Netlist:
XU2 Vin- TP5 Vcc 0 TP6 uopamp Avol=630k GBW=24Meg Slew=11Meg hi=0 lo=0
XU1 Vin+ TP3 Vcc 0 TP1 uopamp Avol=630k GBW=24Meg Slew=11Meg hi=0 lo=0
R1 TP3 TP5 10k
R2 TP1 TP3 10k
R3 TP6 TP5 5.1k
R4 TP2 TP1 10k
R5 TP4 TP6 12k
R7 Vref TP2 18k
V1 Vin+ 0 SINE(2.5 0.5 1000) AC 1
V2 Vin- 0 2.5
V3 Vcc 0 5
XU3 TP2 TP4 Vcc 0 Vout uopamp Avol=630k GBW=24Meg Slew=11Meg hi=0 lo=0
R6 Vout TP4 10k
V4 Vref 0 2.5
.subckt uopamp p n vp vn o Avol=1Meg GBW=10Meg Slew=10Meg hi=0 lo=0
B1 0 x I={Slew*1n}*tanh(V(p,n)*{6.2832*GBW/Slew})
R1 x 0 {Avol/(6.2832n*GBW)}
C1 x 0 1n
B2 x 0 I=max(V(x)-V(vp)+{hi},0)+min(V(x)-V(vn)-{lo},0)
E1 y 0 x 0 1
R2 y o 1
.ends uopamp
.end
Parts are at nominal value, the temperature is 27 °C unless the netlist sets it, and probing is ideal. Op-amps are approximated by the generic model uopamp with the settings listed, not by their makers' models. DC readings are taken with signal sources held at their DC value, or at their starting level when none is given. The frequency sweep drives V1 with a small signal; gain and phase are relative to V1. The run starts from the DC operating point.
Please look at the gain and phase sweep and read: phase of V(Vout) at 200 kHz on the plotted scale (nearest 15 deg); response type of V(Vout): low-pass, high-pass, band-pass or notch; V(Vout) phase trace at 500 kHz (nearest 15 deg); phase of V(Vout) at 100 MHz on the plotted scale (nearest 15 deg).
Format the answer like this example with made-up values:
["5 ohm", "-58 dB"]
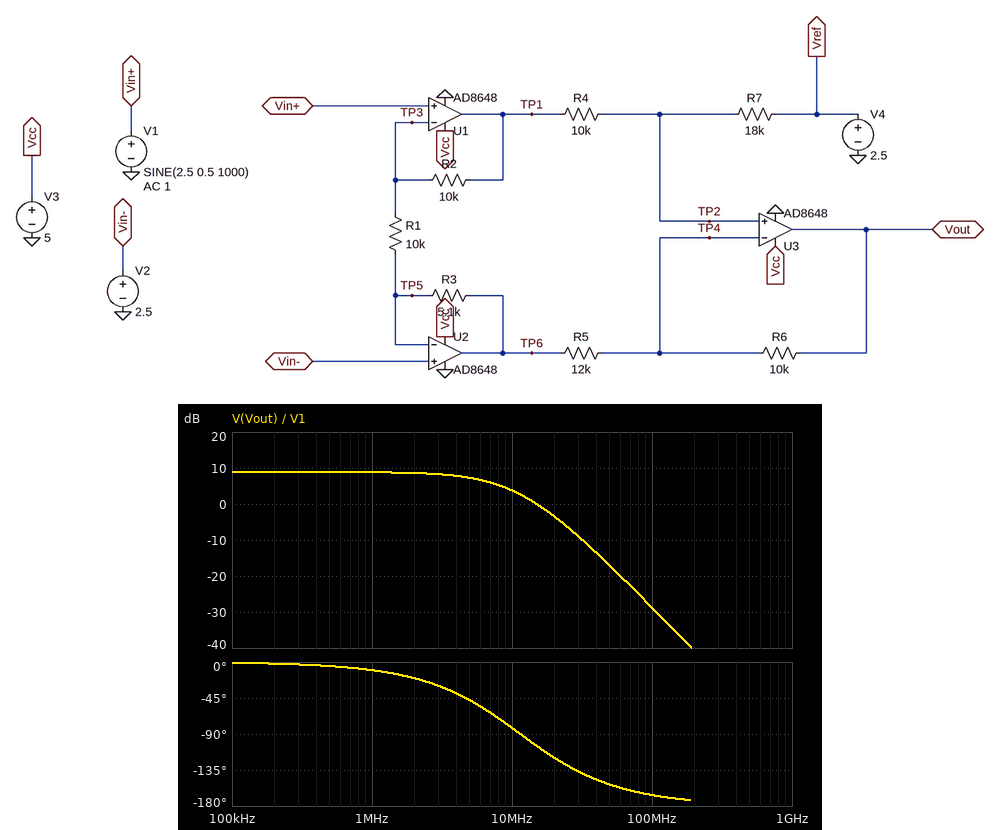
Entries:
["0 deg", "low-pass", "0 deg", "-165 deg"]
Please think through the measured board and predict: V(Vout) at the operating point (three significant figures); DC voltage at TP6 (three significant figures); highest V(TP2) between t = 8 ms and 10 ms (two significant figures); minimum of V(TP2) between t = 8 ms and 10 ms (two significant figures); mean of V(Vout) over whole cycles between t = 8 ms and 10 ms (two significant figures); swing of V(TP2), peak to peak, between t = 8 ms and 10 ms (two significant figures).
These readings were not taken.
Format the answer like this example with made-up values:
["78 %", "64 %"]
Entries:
["2.50 V", "2.50 V", "3.1 V", "1.9 V", "2.5 V", "1.3 V"]
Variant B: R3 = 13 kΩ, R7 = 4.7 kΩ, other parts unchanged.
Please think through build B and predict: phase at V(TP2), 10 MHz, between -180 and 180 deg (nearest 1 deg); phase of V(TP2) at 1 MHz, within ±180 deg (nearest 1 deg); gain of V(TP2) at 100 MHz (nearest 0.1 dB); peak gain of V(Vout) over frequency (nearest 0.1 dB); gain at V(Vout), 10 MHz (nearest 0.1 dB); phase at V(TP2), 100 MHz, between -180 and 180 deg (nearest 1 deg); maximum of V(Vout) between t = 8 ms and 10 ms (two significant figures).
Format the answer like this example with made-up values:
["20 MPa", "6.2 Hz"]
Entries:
["-42 deg", "-6 deg", "-22.5 dB", "7.1 dB", "0.3 dB", "-81 deg", "3.6 V"]
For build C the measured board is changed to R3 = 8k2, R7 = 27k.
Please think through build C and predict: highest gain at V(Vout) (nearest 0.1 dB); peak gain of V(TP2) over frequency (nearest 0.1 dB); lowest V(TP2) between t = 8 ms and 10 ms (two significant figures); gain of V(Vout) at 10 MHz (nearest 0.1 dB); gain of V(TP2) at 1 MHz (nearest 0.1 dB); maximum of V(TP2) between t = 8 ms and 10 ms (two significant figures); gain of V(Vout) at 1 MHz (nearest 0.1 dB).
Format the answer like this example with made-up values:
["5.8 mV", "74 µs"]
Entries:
["10.5 dB", "3.3 dB", "1.8 V", "4.9 dB", "3.2 dB", "3.2 V", "10.4 dB"]
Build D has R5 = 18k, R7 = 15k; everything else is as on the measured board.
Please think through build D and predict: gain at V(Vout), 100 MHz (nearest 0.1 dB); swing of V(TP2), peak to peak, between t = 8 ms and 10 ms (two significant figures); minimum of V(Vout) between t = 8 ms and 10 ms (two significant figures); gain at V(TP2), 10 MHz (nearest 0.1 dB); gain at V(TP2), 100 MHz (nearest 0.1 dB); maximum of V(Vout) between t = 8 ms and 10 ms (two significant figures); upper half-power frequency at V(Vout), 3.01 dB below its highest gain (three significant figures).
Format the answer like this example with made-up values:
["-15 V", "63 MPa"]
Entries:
["-29.4 dB", "1.2 V", "1.4 V", "-1.3 dB", "-17.0 dB", "3.6 V", "7.62 MHz"]
